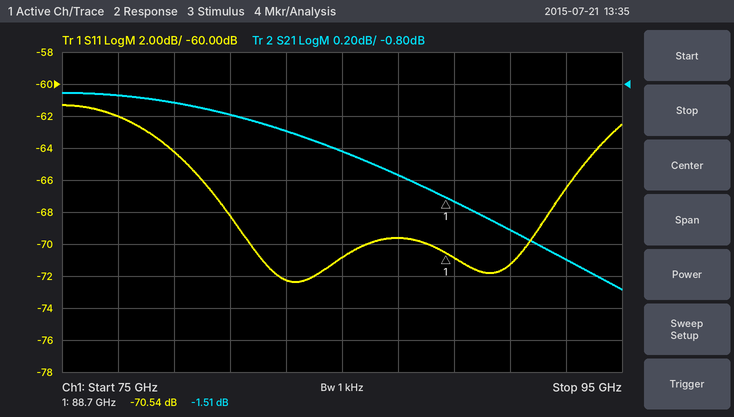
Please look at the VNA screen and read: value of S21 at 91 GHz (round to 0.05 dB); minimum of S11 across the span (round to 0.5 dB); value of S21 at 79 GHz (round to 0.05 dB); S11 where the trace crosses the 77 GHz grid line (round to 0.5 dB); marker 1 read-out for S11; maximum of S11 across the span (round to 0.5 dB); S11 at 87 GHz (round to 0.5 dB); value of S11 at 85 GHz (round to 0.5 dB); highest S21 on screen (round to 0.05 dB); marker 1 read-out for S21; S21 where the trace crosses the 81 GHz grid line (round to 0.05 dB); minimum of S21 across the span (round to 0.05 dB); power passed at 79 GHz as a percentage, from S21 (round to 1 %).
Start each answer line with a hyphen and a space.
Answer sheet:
- -1.70 dB
- -72.5 dB
- -0.90 dB
- -62.0 dB
- -70.54 dB
- -61.5 dB
- -69.5 dB
- -71.0 dB
- -0.85 dB
- -1.51 dB
- -1.00 dB
- -2.10 dB
- 81 %
